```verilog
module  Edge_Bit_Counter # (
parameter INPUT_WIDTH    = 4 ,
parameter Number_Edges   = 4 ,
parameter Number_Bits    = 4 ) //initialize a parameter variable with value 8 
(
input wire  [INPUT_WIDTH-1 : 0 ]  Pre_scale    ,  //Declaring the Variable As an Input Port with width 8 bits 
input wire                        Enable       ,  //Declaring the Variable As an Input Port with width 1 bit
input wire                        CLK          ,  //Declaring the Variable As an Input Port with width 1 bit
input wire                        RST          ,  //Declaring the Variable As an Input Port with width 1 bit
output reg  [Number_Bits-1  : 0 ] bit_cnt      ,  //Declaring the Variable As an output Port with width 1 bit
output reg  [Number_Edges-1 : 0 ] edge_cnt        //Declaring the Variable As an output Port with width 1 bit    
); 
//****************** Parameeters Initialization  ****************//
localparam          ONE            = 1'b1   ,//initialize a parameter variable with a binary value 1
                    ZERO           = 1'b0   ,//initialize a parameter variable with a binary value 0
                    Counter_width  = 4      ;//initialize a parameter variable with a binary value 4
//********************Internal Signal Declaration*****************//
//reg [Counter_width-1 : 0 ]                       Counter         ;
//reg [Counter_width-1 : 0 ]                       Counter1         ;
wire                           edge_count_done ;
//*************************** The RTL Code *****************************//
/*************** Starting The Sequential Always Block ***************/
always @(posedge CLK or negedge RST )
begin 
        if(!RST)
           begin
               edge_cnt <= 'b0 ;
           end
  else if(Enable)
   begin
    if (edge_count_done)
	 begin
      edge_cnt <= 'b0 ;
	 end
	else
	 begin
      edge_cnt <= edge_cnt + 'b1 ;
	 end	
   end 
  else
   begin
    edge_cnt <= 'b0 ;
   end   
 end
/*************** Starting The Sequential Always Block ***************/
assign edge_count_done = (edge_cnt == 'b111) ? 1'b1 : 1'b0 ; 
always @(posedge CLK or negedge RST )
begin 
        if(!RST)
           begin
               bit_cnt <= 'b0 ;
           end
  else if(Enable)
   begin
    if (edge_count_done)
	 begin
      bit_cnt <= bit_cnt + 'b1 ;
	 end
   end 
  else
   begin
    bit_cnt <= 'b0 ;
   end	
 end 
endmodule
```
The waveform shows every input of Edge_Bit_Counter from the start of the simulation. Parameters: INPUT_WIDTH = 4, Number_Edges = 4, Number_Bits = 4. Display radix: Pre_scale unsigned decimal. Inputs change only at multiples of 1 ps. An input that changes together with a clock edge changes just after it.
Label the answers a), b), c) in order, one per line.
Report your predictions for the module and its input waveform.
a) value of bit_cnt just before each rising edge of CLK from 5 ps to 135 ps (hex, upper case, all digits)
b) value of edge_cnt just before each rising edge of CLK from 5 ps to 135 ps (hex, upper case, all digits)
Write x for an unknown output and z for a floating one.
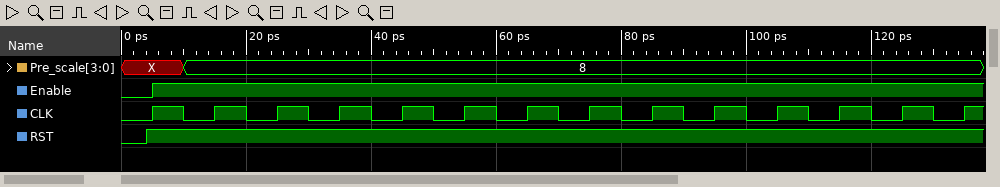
a) 0, 0, 0, 0, 0, 0, 0, 0, 0, 1, 1, 1, 1, 1
b) 0, 0, 1, 2, 3, 4, 5, 6, 7, 0, 1, 2, 3, 4
